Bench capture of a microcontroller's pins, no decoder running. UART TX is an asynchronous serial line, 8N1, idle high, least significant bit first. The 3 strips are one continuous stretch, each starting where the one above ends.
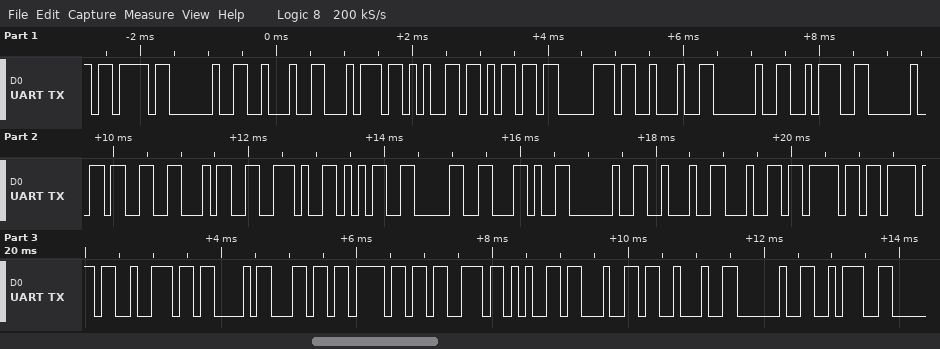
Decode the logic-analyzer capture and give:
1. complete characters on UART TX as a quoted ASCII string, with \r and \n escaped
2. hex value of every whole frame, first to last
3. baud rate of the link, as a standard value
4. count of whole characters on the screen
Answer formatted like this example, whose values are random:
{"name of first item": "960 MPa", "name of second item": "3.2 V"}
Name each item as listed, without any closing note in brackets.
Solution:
{"complete characters on UART TX as a quoted ASCII string, with \\r and \\n escaped": "\"{ \\\"temp\\\" : 34.50, \\\"doorClosed\\\" :\"", "hex value of every whole frame, first to last": "0x7B 0x20 0x22 0x74 0x65 0x6D 0x70 0x22 0x20 0x3A 0x20 0x33 0x34 0x2E 0x35 0x30 0x2C 0x20 0x22 0x64 0x6F 0x6F 0x72 0x43 0x6C 0x6F 0x73 0x65 0x64 0x22 0x20 0x3A", "baud rate of the link, as a standard value": "9600 baud", "count of whole characters on the screen": "32"}
